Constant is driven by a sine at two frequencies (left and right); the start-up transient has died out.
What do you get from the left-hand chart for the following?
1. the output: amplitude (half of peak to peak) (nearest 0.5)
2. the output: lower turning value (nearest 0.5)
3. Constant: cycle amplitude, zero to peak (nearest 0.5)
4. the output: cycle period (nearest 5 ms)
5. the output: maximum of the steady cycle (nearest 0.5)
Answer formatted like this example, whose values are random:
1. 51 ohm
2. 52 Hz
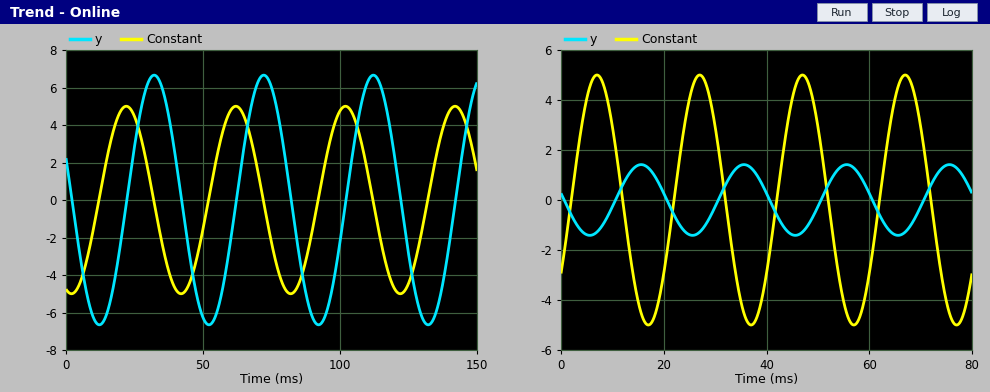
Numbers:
1. 6.5
2. -6.5
3. 5.0
4. 40 ms
5. 6.5
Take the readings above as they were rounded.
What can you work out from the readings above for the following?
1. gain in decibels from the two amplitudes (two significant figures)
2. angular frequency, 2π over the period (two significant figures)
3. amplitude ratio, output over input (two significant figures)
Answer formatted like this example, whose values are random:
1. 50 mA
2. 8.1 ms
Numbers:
1. 2.3 dB
2. 0.16 rad/ms
3. 1.3
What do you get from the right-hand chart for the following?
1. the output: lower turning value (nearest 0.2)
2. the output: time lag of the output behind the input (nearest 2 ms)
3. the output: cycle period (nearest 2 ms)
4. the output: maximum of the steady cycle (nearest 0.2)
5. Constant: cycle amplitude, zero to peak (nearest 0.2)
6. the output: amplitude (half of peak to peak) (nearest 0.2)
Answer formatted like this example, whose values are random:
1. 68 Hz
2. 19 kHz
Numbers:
1. -1.4
2. 8 ms
3. 20 ms
4. 1.4
5. 5.0
6. 1.4
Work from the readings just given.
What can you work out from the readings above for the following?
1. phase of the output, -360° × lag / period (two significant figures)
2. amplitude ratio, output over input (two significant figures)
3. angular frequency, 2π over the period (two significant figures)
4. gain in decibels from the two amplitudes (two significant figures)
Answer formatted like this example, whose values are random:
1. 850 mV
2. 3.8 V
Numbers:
1. -140°
2. 0.28
3. 0.31 rad/ms
4. -11 dB
